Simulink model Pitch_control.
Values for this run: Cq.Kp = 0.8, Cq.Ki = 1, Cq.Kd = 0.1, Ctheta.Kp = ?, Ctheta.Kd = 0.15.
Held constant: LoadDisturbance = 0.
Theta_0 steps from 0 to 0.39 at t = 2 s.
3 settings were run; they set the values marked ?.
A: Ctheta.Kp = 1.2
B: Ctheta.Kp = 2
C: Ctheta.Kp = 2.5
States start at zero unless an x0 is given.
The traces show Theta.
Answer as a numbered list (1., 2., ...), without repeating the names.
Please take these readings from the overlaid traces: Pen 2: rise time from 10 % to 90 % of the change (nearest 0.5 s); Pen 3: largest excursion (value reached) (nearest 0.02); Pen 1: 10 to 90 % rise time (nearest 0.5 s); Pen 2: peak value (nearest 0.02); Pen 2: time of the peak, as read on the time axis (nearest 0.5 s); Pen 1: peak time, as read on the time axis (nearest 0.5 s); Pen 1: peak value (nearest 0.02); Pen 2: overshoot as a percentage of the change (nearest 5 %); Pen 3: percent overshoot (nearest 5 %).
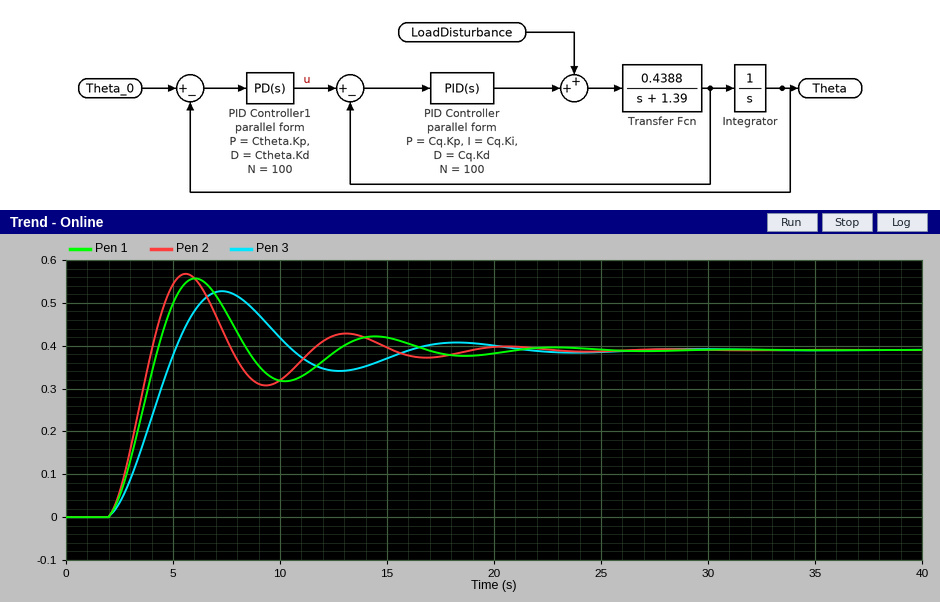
1. 1.5 s
2. 0.52
3. 1.5 s
4. 0.56
5. 5.5 s
6. 6.0 s
7. 0.56
8. 45 %
9. 35 %
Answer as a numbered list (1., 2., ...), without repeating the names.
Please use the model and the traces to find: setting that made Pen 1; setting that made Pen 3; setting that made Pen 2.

1. B
2. A
3. C
